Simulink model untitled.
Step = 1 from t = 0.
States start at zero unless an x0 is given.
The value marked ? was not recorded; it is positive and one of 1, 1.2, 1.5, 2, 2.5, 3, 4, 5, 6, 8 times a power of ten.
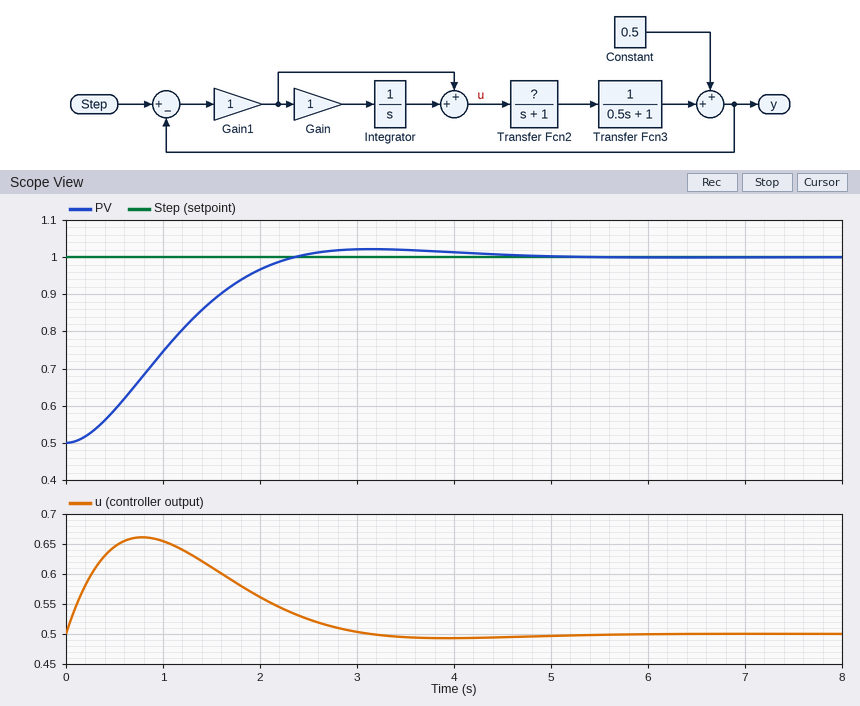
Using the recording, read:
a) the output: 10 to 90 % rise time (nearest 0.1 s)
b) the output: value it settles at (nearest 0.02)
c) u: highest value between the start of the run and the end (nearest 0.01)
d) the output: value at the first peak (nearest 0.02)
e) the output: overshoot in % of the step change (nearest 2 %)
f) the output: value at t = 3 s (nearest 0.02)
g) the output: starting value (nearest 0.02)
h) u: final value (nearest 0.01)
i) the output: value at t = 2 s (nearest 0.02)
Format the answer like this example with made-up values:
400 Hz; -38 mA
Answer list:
1.5 s; 1.00; 0.66; 1.02; 4 %; 1.02; 0.50; 0.50; 0.96
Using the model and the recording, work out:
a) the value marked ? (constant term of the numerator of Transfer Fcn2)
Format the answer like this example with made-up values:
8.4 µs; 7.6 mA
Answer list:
1
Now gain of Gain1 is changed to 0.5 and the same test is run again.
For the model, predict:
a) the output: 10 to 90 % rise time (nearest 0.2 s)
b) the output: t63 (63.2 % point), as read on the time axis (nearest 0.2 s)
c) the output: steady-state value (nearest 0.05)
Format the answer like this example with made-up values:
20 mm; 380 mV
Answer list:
3.4 s; 2.2 s; 1.00
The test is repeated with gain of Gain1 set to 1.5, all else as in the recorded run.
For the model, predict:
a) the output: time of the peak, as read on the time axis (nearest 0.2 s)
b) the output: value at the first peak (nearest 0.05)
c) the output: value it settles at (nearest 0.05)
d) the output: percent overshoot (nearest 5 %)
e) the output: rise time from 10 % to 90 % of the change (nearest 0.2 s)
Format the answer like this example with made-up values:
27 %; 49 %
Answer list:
2.2 s; 1.05; 1.00; 10 %; 1.0 s
